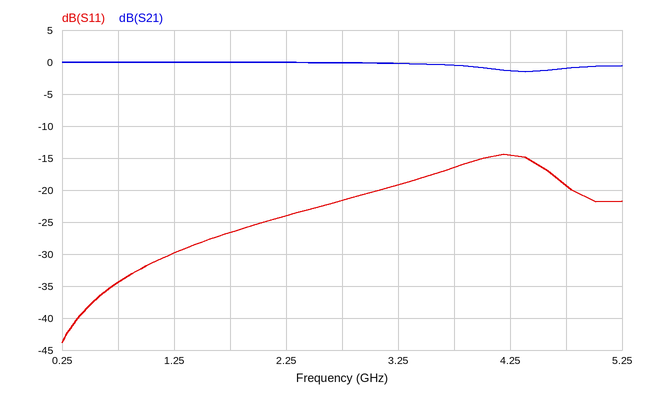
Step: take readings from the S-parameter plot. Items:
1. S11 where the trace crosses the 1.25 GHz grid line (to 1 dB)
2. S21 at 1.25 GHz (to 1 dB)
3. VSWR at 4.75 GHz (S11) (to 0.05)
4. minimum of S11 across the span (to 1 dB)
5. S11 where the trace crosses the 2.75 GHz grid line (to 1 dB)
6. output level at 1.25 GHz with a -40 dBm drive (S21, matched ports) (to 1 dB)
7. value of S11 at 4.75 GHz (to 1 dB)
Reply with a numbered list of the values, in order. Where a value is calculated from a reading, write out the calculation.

1. -30 dB
2. 0 dB
3. |Γ| = 10^(-19/20) = 0.1122; VSWR = (1 + 0.1122)/(1 − 0.1122) ≈ 1.25
4. -44 dB
5. -22 dB
6. -40 dBm + (0 dB) = -40 dBm
7. -19 dB
